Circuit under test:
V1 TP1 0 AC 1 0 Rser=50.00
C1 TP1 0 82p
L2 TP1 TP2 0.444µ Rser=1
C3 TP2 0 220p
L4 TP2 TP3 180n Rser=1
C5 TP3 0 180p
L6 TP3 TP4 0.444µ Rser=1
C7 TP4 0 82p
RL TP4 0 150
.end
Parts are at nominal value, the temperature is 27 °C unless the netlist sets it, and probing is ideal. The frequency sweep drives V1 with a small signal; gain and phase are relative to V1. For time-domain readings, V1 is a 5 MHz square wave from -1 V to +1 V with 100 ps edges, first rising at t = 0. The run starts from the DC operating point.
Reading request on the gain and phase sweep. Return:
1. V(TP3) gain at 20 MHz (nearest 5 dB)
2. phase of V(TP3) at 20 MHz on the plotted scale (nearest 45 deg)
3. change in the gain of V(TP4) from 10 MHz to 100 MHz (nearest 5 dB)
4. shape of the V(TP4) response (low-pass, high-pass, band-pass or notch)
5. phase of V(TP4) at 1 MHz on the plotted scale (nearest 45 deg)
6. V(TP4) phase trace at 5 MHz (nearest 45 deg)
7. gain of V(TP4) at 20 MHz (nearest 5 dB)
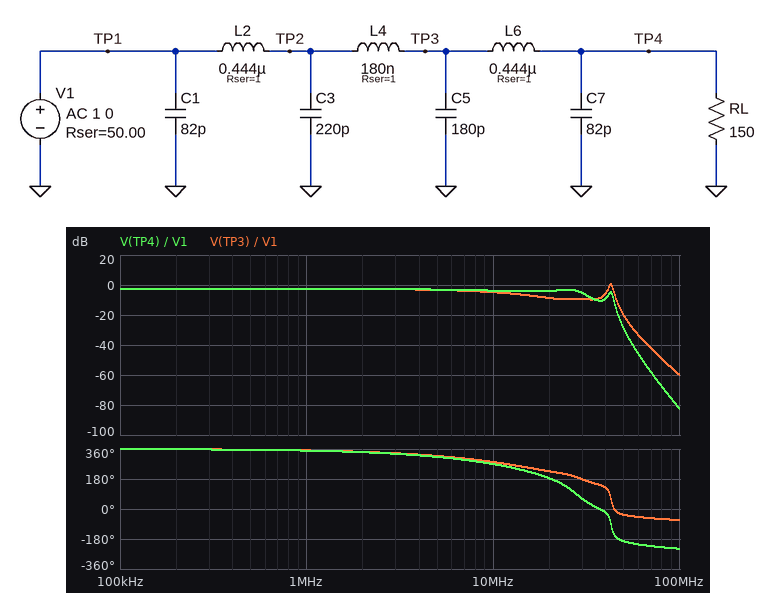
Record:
-10 dB
225 deg
-80 dB
low-pass
360 deg
315 deg
-5 dB
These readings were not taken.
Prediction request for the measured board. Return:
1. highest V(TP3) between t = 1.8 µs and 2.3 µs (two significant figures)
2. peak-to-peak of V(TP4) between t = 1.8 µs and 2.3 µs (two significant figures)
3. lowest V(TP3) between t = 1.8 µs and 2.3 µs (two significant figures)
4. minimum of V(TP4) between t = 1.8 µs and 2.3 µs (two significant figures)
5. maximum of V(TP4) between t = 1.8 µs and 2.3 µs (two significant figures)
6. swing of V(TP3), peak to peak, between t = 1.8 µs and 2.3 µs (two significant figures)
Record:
800 mV
1.6 V
-800 mV
-820 mV
820 mV
1.6 V
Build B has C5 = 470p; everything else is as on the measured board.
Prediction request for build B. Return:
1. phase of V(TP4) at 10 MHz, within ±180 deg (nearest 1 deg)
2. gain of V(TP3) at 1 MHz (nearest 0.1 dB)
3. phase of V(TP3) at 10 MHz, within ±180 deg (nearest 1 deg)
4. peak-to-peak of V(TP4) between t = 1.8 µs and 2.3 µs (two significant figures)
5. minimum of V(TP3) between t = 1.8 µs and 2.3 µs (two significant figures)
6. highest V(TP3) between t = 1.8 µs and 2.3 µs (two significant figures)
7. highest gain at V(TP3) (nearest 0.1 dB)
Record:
-110 deg
-2.7 dB
-97 deg
1.5 V
-750 mV
750 mV
-2.6 dB
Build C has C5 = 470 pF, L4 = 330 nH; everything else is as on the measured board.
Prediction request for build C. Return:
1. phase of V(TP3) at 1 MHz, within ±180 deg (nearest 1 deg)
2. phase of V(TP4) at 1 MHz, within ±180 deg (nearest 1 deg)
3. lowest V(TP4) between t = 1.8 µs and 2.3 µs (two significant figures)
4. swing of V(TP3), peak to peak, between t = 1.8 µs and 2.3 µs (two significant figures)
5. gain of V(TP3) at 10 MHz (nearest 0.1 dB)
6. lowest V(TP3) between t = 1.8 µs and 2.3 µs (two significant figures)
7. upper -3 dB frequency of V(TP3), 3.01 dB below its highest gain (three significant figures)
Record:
-13 deg
-14 deg
-780 mV
1.5 V
-6.8 dB
-740 mV
7.63 MHz
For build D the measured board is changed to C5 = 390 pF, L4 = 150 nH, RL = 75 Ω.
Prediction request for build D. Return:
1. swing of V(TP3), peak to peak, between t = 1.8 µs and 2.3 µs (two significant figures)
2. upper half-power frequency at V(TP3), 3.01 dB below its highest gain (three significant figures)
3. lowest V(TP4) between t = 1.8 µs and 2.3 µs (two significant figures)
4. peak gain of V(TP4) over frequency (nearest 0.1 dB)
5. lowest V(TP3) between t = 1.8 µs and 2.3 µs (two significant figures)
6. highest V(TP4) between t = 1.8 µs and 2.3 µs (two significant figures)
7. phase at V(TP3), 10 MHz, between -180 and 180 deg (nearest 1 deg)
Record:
1.2 V
39.7 MHz
-600 mV
-4.6 dB
-620 mV
600 mV
-82 deg
